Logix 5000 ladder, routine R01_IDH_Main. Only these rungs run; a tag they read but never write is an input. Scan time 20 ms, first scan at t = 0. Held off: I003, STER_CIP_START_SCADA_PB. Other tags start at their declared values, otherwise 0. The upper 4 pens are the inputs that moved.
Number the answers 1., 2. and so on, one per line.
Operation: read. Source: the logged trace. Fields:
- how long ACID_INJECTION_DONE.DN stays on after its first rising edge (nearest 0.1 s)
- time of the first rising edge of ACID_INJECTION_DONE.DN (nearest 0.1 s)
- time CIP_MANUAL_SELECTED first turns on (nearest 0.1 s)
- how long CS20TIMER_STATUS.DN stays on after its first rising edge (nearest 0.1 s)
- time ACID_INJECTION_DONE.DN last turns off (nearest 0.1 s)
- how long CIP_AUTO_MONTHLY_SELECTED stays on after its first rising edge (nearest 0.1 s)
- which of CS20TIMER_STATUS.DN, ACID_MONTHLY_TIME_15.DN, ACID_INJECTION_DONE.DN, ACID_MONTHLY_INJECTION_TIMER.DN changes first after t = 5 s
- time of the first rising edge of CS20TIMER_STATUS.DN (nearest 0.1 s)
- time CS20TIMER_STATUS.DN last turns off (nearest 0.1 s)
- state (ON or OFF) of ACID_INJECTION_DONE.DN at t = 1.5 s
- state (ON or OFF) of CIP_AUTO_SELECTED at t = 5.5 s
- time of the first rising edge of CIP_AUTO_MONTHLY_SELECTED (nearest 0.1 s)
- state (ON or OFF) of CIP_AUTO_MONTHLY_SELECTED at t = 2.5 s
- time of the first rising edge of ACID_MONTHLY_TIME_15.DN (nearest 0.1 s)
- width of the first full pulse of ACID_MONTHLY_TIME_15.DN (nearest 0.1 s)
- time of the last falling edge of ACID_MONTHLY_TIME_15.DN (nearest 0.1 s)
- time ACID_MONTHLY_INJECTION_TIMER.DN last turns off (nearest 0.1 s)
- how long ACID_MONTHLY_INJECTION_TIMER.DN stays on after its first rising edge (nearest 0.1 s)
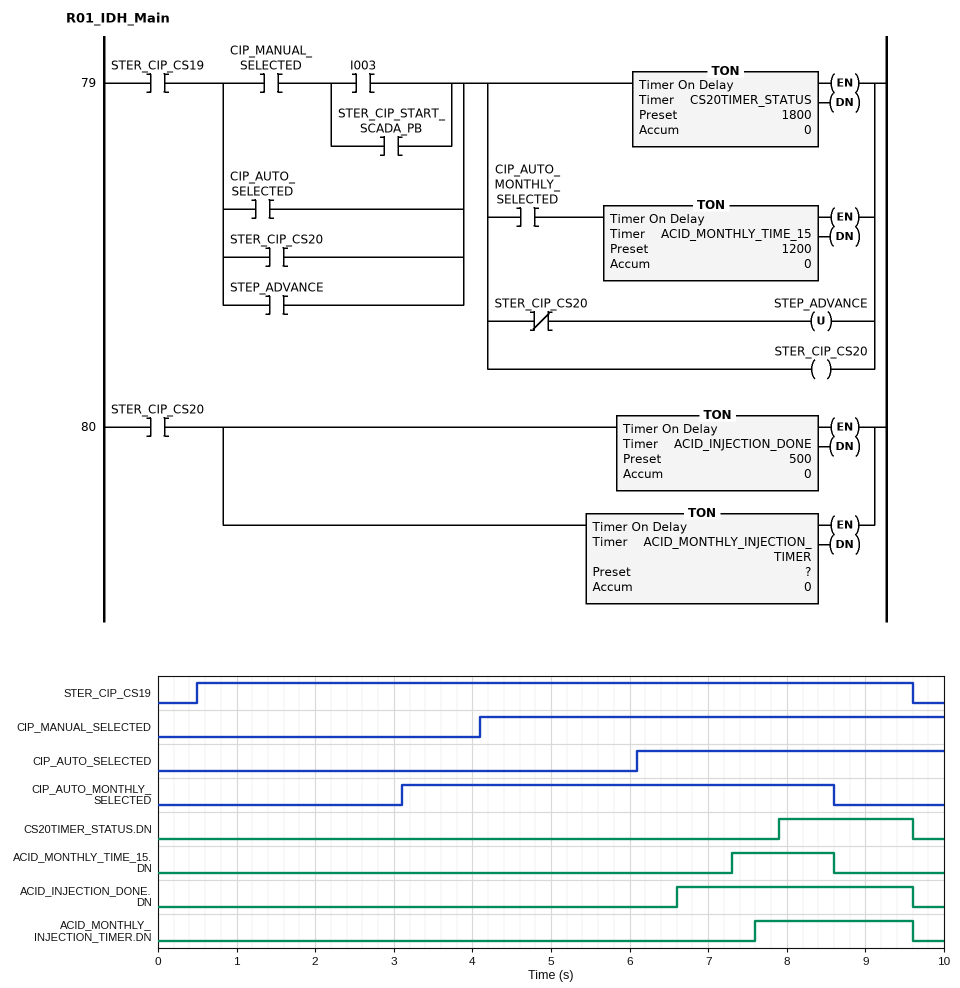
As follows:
1. 3.0 s
2. 6.6 s
3. 4.1 s
4. 1.7 s
5. 9.6 s
6. 5.5 s
7. ACID_INJECTION_DONE.DN
8. 7.9 s
9. 9.6 s
10. OFF
11. OFF
12. 3.1 s
13. OFF
14. 7.3 s
15. 1.3 s
16. 8.6 s
17. 9.6 s
18. 2.0 s
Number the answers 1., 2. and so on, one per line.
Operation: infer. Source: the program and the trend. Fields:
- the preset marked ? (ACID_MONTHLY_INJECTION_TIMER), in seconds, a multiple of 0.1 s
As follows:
1. 1.5 s
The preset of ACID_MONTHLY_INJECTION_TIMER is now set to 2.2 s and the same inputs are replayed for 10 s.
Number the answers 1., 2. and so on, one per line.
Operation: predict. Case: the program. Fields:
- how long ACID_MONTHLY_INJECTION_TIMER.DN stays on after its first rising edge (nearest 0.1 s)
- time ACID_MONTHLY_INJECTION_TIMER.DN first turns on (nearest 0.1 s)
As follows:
1. 1.3 s
2. 8.3 s
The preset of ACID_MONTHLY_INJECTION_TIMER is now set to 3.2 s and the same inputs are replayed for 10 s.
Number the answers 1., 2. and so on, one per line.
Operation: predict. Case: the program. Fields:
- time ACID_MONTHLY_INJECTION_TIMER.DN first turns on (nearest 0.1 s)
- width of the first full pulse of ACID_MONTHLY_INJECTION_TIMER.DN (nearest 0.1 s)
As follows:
1. 9.3 s
2. 0.3 s
